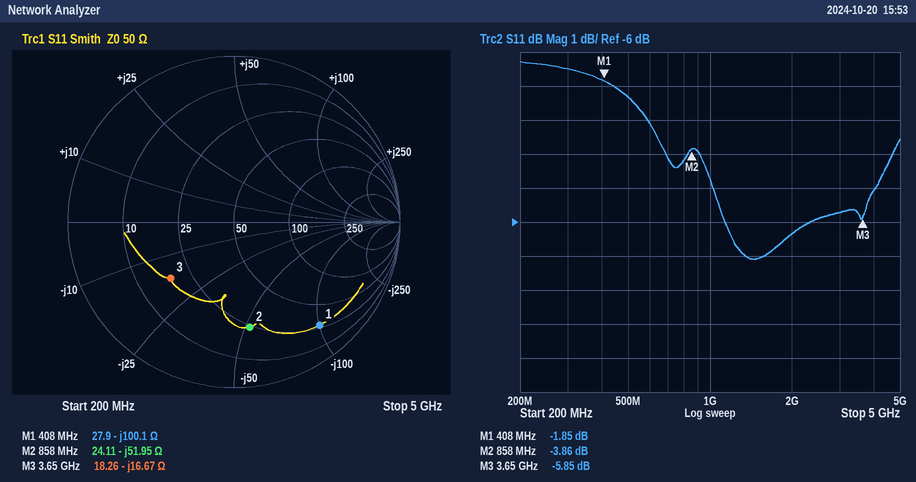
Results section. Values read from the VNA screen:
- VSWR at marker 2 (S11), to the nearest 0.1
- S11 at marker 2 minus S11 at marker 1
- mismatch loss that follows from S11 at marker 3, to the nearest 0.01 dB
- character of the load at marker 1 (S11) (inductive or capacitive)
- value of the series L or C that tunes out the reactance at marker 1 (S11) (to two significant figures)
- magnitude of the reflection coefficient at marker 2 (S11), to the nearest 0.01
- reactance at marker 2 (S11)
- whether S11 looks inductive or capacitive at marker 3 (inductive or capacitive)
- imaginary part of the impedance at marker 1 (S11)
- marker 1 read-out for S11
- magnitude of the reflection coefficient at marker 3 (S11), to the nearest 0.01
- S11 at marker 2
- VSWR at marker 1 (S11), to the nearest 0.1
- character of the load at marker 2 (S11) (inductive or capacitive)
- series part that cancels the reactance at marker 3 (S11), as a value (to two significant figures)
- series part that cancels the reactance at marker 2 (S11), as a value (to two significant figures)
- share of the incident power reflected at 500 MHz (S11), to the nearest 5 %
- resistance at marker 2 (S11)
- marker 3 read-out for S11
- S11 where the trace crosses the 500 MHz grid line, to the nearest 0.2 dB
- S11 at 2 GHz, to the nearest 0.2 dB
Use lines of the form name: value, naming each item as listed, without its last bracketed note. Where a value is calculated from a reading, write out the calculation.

VSWR at marker 2 (S11), to the nearest 0.1: (1 + 0.6412)/(1 − 0.6412) ≈ 4.6
S11 at marker 2 minus S11 at marker 1: -3.86 − (-1.85) = -2.01 dB
mismatch loss that follows from S11 at marker 3, to the nearest 0.01 dB: −10 log10(1 − 10^(-5.85/10)) ≈ 1.31 dB
character of the load at marker 1 (S11): capacitive
value of the series L or C that tunes out the reactance at marker 1 (S11): L = 100.1 Ω/(2π × 408 MHz) ≈ 39 nH
magnitude of the reflection coefficient at marker 2 (S11), to the nearest 0.01: 0.64
reactance at marker 2: -51.95 Ω
whether S11 looks inductive or capacitive at marker 3: capacitive
imaginary part of the impedance at marker 1: -100.1 Ω
marker 1 read-out for S11: -1.85 dB
magnitude of the reflection coefficient at marker 3 (S11), to the nearest 0.01: 0.51
S11 at marker 2: -3.86 dB
VSWR at marker 1 (S11), to the nearest 0.1: (1 + 0.8082)/(1 − 0.8082) ≈ 9.4
character of the load at marker 2 (S11): capacitive
series part that cancels the reactance at marker 3 (S11), as a value: L = 16.67 Ω/(2π × 3.65 GHz) ≈ 727 pH, so 730 pH to two significant figures
series part that cancels the reactance at marker 2 (S11), as a value: L = 51.95 Ω/(2π × 858 MHz) ≈ 9.6 nH
share of the incident power reflected at 500 MHz (S11), to the nearest 5 %: 10^(-2.4/10) ≈ 57.5 %, so 60 % to the nearest 5 %
resistance at marker 2: 24.11 Ω
marker 3 read-out for S11: -5.85 dB
S11 where the trace crosses the 500 MHz grid line, to the nearest 0.2 dB: -2.4 dB
S11 at 2 GHz, to the nearest 0.2 dB: -6.4 dB
